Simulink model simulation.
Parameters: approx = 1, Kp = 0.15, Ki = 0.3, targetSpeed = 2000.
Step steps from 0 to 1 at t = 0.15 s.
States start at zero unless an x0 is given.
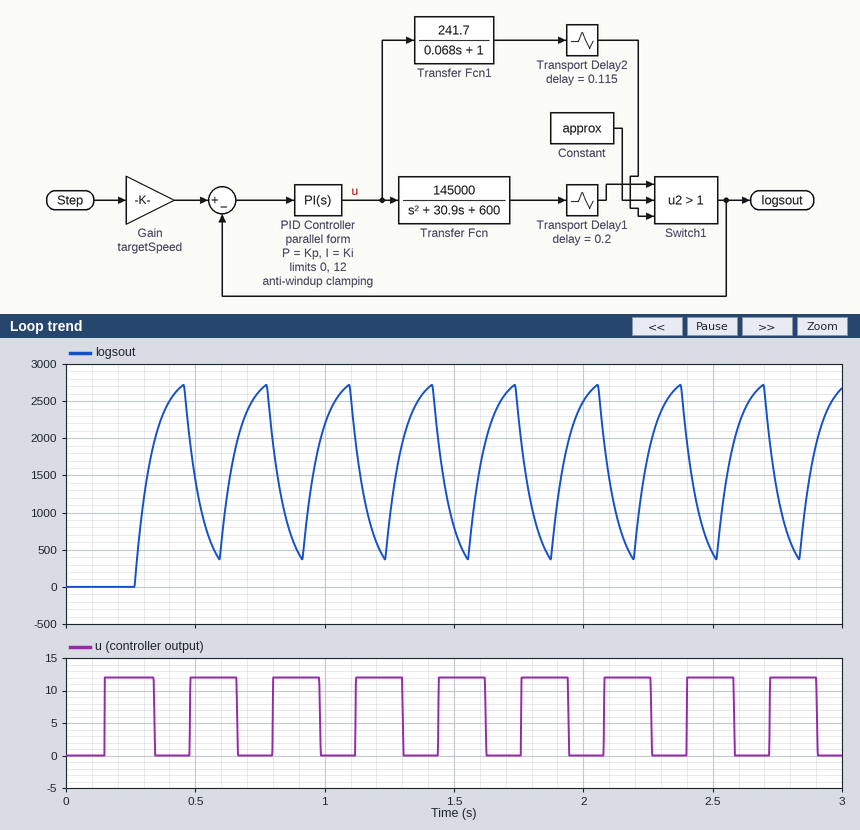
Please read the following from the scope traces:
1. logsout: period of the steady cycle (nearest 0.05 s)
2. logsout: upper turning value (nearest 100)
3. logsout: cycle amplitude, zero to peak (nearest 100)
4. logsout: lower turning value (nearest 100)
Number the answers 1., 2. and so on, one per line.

1. 0.30 s
2. 2700
3. 1200
4. 400
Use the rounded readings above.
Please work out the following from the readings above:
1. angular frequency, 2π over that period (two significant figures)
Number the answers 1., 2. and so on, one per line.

1. 21 rad/s
